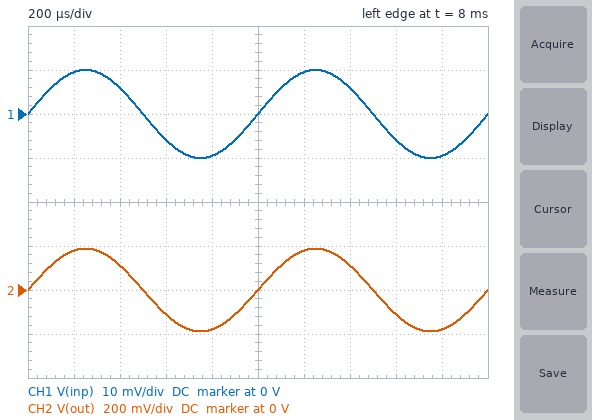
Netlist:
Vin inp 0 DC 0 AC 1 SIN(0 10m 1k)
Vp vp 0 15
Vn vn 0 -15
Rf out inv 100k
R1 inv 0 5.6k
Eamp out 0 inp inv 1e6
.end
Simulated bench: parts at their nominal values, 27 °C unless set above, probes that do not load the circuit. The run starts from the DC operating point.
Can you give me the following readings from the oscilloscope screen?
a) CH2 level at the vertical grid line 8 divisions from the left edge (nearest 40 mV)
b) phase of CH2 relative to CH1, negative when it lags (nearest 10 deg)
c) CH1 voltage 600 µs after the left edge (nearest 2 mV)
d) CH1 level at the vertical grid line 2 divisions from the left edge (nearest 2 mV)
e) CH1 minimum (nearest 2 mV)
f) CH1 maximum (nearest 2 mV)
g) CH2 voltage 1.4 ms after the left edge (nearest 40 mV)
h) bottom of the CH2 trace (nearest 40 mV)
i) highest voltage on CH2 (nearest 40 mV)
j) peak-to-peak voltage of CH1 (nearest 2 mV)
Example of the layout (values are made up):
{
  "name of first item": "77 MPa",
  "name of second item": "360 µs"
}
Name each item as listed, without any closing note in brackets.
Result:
{
  "CH2 level at the vertical grid line 8 divisions from the left edge": "-120 mV",
  "phase of CH2 relative to CH1, negative when it lags": "0 deg",
  "CH1 voltage 600 µs after the left edge": "-6 mV",
  "CH1 level at the vertical grid line 2 divisions from the left edge": "6 mV",
  "CH1 minimum": "-10 mV",
  "CH1 maximum": "10 mV",
  "CH2 voltage 1.4 ms after the left edge": "120 mV",
  "bottom of the CH2 trace": "-200 mV",
  "highest voltage on CH2": "200 mV",
  "peak-to-peak voltage of CH1": "20 mV"
}
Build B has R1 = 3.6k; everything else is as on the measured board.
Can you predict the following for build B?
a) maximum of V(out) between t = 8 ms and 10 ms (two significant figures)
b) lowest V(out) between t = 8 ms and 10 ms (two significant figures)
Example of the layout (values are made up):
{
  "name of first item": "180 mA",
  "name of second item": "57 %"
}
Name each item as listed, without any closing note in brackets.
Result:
{
  "maximum of V(out) between t = 8 ms and 10 ms": "290 mV",
  "lowest V(out) between t = 8 ms and 10 ms": "-290 mV"
}
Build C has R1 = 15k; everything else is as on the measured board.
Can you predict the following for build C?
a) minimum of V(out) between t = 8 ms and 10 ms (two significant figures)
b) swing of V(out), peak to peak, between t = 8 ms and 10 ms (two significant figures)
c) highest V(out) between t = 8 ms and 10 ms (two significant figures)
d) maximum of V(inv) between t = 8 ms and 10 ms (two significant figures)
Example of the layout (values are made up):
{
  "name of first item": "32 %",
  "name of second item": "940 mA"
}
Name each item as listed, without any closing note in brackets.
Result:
{
  "minimum of V(out) between t = 8 ms and 10 ms": "-77 mV",
  "swing of V(out), peak to peak, between t = 8 ms and 10 ms": "150 mV",
  "highest V(out) between t = 8 ms and 10 ms": "77 mV",
  "maximum of V(inv) between t = 8 ms and 10 ms": "10 mV"
}
